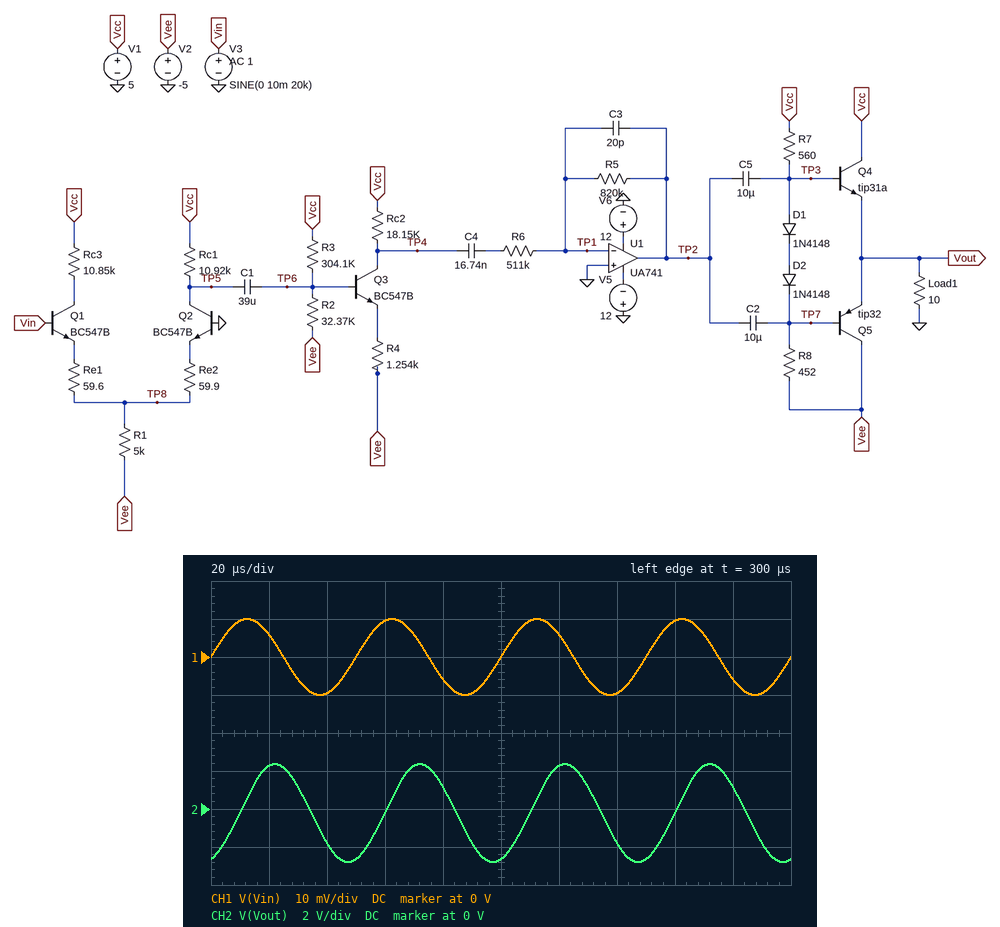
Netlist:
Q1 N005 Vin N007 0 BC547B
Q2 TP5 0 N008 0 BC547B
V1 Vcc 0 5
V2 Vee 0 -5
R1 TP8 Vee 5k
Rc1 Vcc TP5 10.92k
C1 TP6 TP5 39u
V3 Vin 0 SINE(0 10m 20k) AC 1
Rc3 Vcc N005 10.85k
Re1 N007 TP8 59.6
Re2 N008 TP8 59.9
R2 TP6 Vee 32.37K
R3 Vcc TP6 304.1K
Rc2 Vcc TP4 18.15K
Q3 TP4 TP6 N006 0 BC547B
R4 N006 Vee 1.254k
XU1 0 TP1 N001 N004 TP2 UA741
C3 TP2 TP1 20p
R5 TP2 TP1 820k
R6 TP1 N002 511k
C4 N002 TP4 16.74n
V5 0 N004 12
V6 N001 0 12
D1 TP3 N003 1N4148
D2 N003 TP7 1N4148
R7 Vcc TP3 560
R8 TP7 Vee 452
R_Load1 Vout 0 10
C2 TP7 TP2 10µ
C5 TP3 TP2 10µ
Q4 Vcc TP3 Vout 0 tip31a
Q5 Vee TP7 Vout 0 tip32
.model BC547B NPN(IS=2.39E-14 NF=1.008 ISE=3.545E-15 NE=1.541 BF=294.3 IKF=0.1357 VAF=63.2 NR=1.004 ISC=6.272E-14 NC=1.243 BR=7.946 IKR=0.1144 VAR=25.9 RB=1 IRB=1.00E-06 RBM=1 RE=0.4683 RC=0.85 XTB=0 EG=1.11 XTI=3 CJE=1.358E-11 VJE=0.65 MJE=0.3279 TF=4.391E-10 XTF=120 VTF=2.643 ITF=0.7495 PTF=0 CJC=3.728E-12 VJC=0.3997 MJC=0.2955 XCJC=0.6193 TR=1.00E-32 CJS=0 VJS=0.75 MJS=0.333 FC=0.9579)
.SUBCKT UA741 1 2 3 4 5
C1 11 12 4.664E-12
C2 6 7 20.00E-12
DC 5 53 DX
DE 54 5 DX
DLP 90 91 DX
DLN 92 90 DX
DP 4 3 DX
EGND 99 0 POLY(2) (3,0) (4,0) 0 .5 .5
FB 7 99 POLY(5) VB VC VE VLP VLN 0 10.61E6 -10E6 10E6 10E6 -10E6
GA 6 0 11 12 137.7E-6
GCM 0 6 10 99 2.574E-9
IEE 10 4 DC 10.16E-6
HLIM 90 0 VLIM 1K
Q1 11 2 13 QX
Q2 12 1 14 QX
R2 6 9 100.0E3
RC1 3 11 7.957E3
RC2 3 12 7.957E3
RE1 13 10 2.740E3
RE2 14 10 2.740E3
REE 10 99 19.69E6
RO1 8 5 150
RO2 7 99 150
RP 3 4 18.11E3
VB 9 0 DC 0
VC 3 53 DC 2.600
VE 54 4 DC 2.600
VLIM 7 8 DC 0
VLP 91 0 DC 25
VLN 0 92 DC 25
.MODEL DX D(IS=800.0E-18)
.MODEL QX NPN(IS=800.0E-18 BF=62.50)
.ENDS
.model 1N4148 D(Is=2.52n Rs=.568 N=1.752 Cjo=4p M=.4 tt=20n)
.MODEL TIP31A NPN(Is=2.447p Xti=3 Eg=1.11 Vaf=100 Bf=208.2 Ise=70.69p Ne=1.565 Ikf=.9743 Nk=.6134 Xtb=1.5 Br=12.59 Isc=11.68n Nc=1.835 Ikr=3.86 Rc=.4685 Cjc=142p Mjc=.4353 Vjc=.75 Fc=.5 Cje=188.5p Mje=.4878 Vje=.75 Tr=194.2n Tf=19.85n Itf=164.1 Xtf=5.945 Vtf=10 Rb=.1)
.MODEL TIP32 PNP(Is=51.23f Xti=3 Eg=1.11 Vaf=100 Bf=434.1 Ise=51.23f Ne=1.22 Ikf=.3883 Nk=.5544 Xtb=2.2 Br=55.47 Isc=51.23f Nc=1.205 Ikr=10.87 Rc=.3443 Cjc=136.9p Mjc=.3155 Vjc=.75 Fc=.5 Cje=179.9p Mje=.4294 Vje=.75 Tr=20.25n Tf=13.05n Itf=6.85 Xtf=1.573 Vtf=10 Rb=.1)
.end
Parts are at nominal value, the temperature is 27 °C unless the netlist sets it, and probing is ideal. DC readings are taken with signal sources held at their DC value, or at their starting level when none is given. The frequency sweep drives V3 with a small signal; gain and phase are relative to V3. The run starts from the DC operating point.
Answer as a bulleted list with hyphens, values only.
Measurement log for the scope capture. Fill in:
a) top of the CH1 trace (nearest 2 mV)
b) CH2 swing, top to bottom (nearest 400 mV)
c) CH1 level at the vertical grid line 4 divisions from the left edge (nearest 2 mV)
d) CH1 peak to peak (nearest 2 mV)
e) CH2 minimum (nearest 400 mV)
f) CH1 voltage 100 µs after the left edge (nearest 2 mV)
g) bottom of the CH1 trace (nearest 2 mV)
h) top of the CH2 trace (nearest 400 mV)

- 10 mV
- 5.2 V
- -6 mV
- 20 mV
- -2.8 V
- 0 V
- -10 mV
- 2.4 V
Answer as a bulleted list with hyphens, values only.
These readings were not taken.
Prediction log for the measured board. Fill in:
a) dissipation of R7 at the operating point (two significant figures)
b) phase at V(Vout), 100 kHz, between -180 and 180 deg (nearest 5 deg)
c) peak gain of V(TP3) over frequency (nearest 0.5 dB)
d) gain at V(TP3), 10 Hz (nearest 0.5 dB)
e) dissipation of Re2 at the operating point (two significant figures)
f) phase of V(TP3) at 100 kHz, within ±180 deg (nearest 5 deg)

- 39 mW
- -105 deg
- 56.0 dB
- 37.5 dB
- 11 µW
- -105 deg
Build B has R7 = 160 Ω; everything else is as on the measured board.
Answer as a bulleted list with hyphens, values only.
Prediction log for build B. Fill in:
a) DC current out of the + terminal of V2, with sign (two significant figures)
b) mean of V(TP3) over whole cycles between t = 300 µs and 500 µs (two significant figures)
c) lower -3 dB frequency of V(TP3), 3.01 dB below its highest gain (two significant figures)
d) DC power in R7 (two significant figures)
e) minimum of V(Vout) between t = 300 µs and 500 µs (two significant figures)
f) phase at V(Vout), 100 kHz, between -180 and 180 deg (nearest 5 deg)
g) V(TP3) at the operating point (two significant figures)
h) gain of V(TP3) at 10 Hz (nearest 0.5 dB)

- -130 mA
- 2.6 V
- 79 Hz
- 38 mW
- -400 mV
- -105 deg
- 2.5 V
- 32.0 dB
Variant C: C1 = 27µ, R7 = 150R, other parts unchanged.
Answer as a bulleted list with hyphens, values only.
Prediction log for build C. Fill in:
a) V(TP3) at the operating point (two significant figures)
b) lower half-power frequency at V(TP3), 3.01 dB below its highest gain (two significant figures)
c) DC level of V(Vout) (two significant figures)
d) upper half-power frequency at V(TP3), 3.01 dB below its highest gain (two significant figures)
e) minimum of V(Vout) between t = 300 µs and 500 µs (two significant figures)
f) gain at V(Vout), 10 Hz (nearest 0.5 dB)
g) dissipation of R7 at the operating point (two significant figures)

- 2.6 V
- 82 Hz
- 2.0 V
- 9.5 kHz
- -270 mV
- 31.5 dB
- 37 mW
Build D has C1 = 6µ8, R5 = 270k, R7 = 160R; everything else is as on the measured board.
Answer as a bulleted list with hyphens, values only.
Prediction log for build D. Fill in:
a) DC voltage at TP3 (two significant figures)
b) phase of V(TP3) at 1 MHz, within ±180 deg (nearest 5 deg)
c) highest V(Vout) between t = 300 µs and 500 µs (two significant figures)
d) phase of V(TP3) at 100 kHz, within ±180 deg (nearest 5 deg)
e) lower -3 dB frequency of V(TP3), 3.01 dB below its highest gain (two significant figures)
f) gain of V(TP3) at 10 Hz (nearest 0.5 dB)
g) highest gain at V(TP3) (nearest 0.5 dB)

- 2.5 V
- 75 deg
- 3.6 V
- -95 deg
- 80 Hz
- 22.5 dB
- 46.5 dB
